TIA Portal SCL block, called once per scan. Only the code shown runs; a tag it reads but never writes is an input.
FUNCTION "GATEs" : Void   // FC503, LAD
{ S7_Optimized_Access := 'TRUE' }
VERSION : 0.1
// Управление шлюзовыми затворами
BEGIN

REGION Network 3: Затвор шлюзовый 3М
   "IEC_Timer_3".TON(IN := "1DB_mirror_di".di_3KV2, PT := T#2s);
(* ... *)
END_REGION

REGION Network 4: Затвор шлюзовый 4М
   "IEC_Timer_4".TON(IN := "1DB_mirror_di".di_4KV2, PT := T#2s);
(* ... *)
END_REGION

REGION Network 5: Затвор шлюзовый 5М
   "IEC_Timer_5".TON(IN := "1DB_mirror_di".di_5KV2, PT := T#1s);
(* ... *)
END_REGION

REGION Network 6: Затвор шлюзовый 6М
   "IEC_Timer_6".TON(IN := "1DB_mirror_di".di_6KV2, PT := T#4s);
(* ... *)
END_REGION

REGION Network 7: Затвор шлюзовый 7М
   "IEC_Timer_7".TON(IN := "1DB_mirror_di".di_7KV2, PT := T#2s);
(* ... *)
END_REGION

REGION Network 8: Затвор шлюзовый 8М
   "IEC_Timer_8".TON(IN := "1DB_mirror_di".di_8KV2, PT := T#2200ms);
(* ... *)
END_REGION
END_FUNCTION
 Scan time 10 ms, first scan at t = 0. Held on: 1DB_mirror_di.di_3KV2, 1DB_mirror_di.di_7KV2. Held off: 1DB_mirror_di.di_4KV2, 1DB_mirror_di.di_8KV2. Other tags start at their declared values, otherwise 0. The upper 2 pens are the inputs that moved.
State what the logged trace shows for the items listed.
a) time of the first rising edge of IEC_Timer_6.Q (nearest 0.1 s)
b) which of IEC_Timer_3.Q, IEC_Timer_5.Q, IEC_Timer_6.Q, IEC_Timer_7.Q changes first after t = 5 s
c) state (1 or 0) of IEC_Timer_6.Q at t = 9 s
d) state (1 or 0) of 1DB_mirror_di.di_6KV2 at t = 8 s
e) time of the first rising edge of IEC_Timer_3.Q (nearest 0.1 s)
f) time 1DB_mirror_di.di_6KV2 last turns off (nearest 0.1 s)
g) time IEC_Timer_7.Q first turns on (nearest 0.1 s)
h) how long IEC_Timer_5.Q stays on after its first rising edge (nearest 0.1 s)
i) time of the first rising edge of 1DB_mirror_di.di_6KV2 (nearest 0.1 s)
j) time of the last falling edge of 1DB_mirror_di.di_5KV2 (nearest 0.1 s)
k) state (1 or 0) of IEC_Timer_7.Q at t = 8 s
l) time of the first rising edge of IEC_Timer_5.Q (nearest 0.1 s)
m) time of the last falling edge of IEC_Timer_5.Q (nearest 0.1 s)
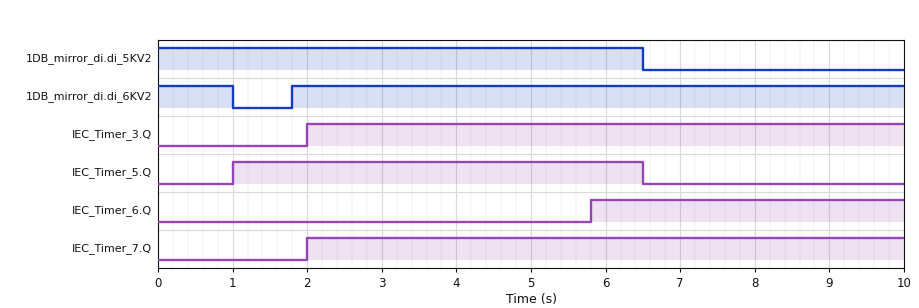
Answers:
5.8 s
IEC_Timer_6.Q
1
1
2.0 s
1.0 s
2.0 s
5.5 s
1.8 s
6.5 s
1
1.0 s
6.5 s
